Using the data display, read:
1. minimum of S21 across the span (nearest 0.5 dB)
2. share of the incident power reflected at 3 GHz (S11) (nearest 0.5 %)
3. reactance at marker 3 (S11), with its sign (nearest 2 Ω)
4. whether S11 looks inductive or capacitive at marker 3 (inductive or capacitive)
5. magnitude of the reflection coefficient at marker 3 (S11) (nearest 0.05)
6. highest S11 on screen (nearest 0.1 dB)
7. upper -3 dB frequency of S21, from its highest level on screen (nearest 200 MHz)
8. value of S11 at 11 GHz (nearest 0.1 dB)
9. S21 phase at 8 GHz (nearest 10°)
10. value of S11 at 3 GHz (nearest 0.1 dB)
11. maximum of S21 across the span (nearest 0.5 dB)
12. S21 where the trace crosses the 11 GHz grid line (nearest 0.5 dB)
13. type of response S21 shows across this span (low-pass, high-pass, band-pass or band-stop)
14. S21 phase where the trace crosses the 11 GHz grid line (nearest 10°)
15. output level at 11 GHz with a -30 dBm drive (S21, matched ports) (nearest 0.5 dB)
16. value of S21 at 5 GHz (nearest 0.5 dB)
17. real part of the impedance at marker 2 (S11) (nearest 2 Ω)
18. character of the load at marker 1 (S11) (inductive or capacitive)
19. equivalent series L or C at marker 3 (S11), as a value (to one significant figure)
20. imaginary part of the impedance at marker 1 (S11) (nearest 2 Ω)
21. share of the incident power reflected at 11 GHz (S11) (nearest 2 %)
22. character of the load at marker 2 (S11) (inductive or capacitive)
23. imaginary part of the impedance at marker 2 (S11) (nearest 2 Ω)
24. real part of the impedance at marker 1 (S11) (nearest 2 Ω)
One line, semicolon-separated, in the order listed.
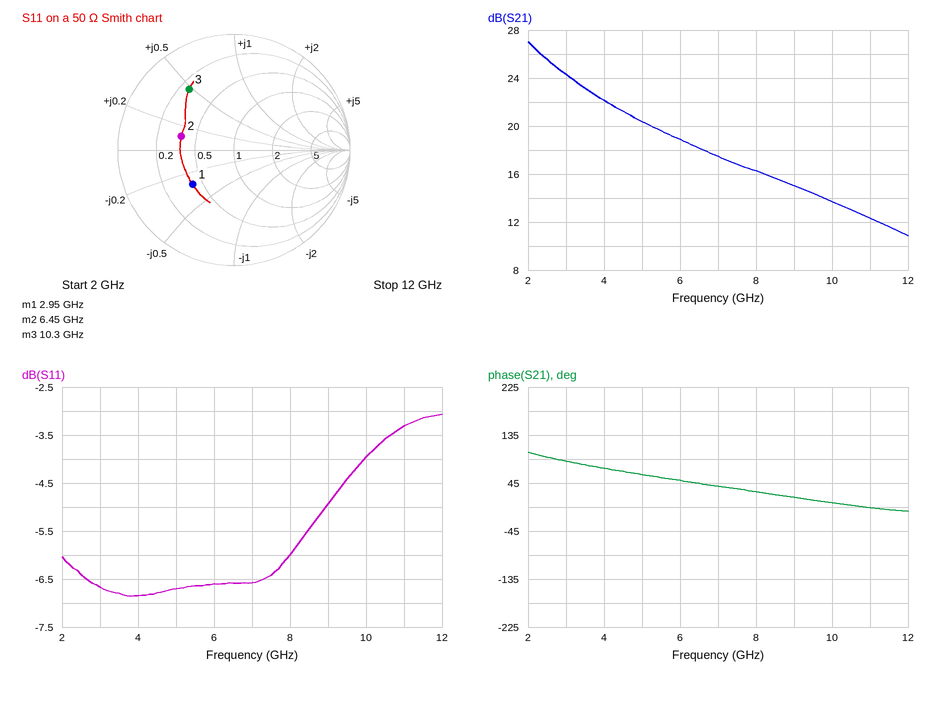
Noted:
11.0 dB; 21.5 %; +24 Ω; inductive; 0.65; -3.1 dB; 3.2 GHz; -3.3 dB; 30°; -6.7 dB; 27.0 dB; 12.5 dB; low-pass; 0°; -17.5 dBm; 20.5 dB; 18 Ω; capacitive; 400 pH; -16 Ω; 46 %; inductive; +6 Ω; 20 Ω
